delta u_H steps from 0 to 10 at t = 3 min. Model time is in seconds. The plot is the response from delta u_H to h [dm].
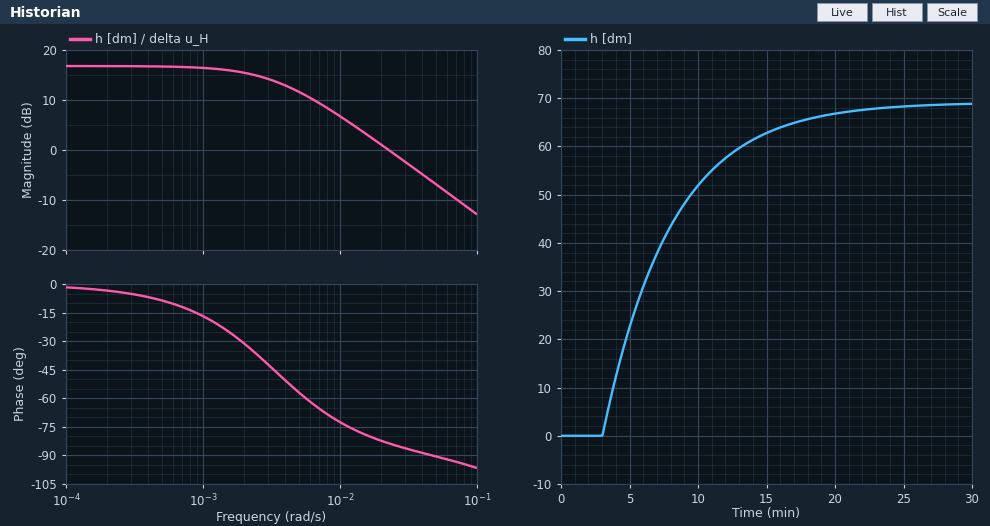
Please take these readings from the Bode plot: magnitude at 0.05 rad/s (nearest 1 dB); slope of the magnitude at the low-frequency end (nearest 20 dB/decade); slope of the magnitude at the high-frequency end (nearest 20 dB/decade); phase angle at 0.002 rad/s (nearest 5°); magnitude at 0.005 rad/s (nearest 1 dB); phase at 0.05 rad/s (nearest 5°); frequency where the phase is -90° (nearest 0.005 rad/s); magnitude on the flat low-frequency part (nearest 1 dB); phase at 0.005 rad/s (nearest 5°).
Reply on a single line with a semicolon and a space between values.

-7 dB; 0 dB/decade; -20 dB/decade; -30°; 12 dB; -90°; 0.045 rad/s; 17 dB; -55°
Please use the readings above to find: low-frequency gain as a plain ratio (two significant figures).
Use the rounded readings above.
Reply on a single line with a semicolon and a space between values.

7.1
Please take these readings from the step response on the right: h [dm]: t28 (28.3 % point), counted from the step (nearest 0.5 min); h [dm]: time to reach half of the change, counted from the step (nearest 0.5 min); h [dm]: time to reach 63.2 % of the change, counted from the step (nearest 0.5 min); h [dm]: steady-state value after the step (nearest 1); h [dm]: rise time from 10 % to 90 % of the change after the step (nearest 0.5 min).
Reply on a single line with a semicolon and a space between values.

1.5 min; 3.5 min; 5.0 min; 69; 11.0 min
